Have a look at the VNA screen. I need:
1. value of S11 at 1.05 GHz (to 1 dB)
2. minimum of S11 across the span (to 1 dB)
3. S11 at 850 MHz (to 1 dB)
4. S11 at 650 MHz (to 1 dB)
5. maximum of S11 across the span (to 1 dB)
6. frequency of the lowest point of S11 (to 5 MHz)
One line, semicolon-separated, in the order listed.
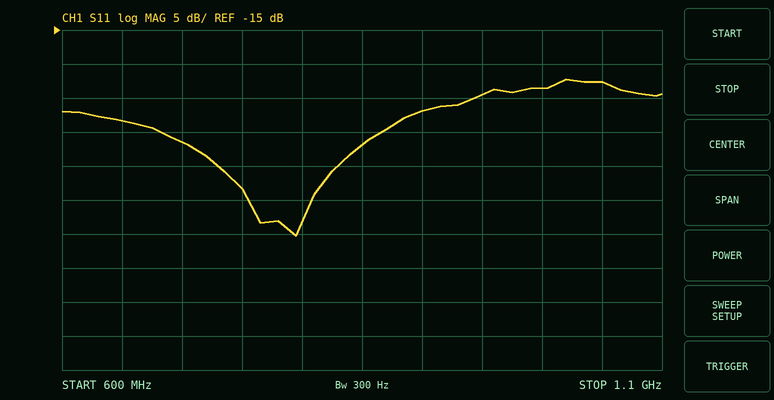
-23 dB; -45 dB; -32 dB; -28 dB; -22 dB; 795 MHz
